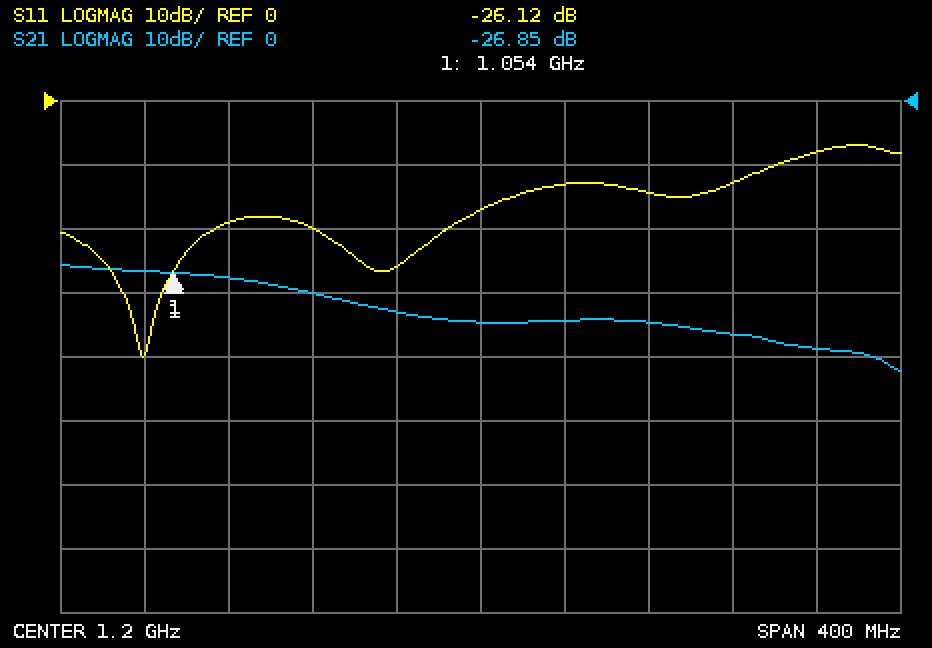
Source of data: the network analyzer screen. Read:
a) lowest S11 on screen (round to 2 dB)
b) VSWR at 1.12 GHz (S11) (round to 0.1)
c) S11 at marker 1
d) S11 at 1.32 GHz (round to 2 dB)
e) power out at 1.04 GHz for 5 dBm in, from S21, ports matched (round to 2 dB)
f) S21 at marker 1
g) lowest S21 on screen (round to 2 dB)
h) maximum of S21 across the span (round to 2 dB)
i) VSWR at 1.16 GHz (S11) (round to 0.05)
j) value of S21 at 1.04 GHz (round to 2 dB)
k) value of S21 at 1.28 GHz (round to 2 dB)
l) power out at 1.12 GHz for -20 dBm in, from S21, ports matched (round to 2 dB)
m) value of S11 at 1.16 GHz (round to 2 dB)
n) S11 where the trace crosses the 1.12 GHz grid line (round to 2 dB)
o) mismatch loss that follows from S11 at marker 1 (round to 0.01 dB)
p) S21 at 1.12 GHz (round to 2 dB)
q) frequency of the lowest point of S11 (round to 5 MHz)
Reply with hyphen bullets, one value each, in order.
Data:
- -40 dB
- 1.2
- -26.12 dB
- -12 dB
- -22 dBm
- -26.85 dB
- -42 dB
- -26 dB
- 1.10
- -26 dB
- -34 dB
- -50 dBm
- -26 dB
- -20 dB
- 0.01 dB
- -30 dB
- 1.040 GHz
